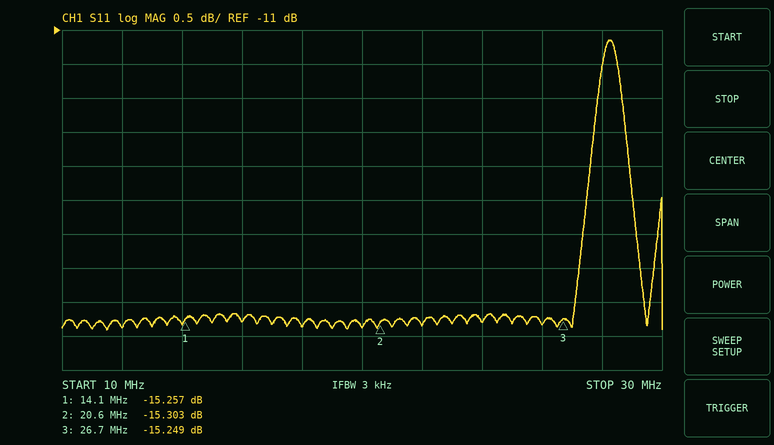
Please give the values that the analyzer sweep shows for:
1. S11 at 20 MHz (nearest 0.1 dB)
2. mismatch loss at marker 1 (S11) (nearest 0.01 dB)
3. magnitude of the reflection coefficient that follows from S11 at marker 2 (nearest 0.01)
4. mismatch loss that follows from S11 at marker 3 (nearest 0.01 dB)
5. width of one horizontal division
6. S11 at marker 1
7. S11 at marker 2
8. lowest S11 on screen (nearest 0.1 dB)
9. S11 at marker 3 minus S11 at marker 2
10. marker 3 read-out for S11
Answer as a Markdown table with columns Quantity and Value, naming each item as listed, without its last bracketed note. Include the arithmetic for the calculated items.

| Quantity | Value |
|---|---|
| S11 at 20 MHz | -15.4 dB |
| mismatch loss at marker 1 (S11) | −10 log10(1 − 10^(-15.257/10)) ≈ 0.13 dB |
| magnitude of the reflection coefficient that follows from S11 at marker 2 | 10^(-15.303/20) ≈ 0.17 |
| mismatch loss that follows from S11 at marker 3 | −10 log10(1 − 10^(-15.249/10)) ≈ 0.13 dB |
| width of one horizontal division | 2 MHz |
| S11 at marker 1 | -15.257 dB |
| S11 at marker 2 | -15.303 dB |
| lowest S11 on screen | -15.4 dB |
| S11 at marker 3 minus S11 at marker 2 | -15.249 − (-15.303) = 0.054 dB |
| marker 3 read-out for S11 | -15.249 dB |
